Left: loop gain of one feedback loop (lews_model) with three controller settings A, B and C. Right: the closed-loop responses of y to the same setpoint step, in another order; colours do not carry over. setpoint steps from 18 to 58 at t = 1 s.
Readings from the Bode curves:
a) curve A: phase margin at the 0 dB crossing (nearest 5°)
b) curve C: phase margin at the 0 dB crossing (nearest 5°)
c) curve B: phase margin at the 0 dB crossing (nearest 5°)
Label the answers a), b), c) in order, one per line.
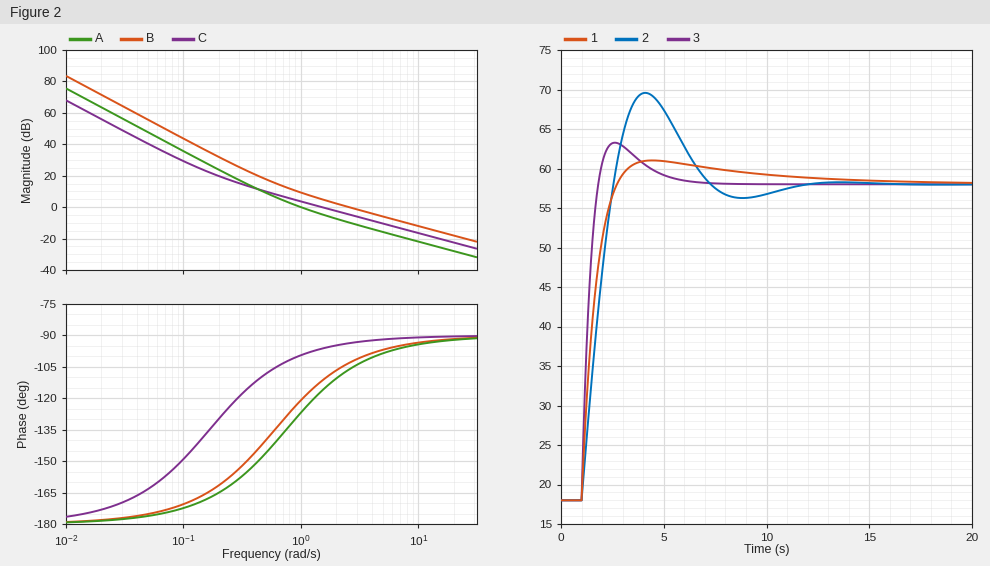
a) 55°
b) 85°
c) 75°
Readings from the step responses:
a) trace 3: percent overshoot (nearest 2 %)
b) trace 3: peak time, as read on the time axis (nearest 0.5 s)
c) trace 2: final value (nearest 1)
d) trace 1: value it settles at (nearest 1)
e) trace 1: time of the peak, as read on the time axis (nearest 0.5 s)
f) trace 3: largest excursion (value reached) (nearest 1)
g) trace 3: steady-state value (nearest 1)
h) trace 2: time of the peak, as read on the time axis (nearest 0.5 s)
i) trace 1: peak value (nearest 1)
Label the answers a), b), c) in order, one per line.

a) 14 %
b) 2.5 s
c) 58
d) 58
e) 4.5 s
f) 63
g) 58
h) 4.0 s
i) 61
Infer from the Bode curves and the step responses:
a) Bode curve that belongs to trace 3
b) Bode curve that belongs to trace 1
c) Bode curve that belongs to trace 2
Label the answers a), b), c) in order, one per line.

a) B
b) C
c) A
